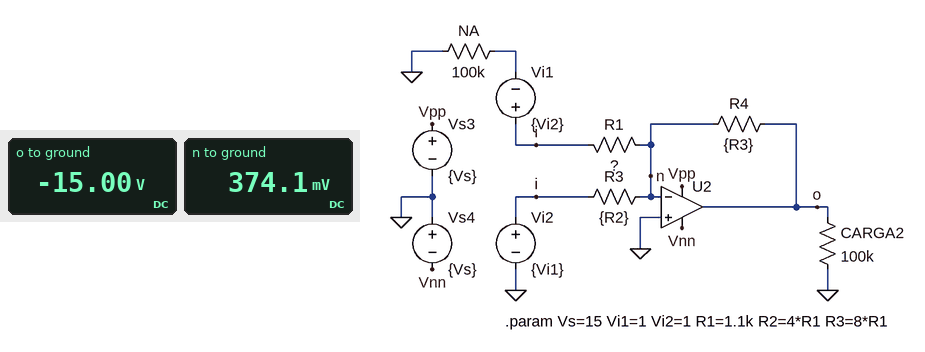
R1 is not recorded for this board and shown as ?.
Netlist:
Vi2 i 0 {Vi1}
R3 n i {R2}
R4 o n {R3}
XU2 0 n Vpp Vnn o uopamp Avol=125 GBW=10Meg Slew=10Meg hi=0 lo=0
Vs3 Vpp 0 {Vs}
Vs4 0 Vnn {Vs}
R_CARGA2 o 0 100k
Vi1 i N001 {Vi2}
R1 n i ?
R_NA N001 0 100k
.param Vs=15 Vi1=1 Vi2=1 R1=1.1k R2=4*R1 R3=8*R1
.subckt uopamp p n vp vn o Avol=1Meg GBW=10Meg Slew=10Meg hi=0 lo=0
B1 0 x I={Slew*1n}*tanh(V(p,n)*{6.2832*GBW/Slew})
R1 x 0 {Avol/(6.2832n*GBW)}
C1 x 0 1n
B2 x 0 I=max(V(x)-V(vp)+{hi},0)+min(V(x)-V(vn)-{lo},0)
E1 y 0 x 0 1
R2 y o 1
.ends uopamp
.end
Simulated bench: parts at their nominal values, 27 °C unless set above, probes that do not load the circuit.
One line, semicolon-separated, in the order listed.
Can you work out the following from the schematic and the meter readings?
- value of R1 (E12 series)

390 Ω
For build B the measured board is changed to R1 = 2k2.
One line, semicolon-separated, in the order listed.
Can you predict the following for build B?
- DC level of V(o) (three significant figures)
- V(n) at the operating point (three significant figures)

-5.67 V; 46.7 mV
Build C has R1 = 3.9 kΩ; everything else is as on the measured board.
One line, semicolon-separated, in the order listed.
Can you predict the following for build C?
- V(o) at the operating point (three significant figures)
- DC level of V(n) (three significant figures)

-4.08 V; 33.1 mV
